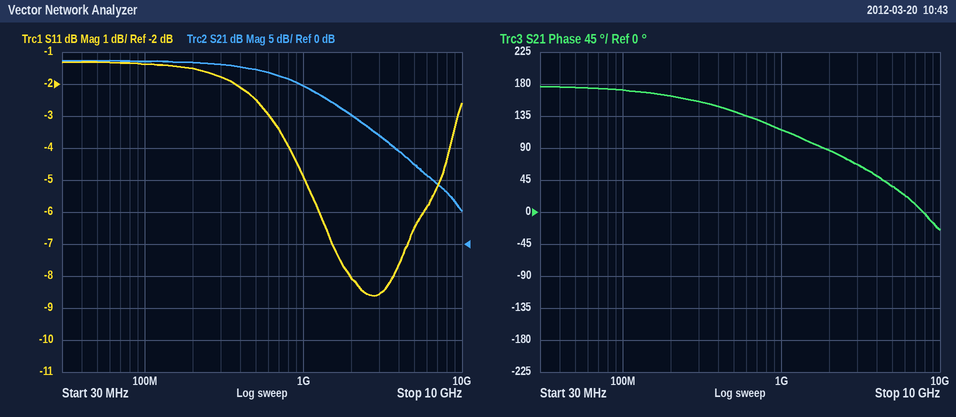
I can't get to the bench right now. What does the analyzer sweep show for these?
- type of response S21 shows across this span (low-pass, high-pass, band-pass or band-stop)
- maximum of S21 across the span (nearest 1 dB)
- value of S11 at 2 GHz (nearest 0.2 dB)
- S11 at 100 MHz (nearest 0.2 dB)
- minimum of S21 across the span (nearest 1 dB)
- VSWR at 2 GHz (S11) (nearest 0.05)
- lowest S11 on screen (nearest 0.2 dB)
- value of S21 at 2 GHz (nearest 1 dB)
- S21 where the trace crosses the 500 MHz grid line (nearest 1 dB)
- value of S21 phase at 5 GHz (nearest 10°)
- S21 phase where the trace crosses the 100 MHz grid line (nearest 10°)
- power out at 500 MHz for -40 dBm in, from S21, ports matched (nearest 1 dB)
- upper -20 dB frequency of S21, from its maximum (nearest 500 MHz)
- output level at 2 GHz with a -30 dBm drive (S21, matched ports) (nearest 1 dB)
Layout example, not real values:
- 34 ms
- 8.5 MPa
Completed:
- low-pass
- 29 dB
- -8.0 dB
- -1.4 dB
- 5 dB
- 2.30
- -8.6 dB
- 20 dB
- 27 dB
- 40°
- 170°
- -13 dBm
- 7.5 GHz
- -10 dBm
